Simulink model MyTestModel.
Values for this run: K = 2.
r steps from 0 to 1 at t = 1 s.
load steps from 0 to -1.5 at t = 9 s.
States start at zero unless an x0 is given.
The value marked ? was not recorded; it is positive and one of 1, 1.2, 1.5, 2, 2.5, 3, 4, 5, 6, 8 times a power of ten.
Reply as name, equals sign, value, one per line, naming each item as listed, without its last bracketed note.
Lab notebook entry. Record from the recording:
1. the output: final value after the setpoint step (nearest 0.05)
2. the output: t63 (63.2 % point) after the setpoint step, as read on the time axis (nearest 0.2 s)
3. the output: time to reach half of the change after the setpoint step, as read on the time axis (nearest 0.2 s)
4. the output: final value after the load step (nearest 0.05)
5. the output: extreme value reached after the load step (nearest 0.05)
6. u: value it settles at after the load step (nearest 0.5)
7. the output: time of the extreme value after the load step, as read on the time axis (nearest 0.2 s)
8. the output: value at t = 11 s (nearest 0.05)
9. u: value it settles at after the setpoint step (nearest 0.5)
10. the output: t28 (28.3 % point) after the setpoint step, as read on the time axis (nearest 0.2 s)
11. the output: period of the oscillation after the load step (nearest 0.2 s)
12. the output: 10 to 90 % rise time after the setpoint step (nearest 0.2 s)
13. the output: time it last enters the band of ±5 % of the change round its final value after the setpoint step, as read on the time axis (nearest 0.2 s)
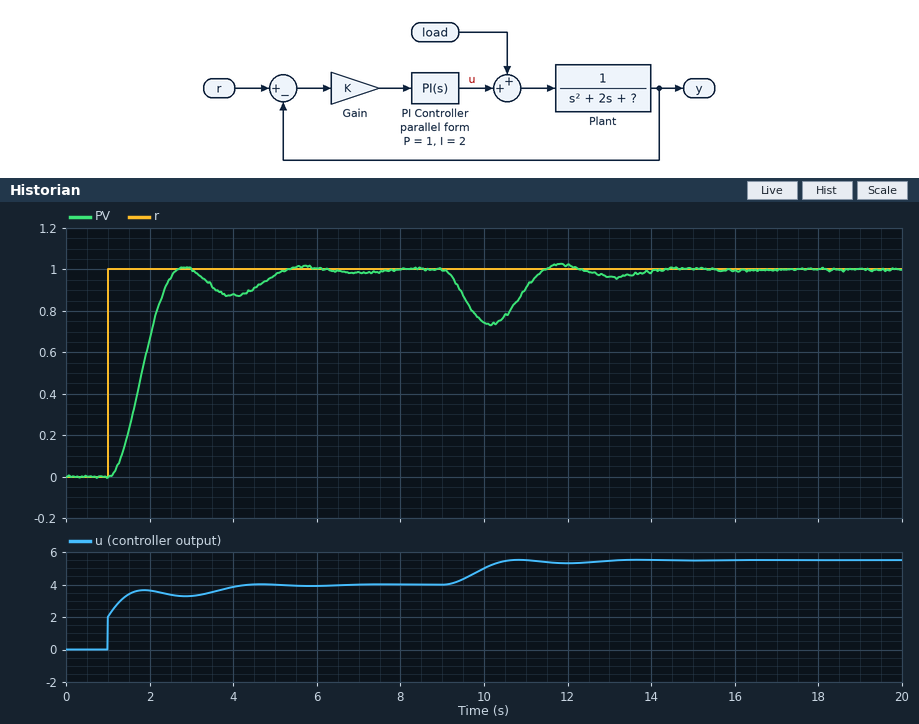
the output: final value after the setpoint step = 1.00
the output: t63 (63.2 % point) after the setpoint step, as read on the time axis = 2.0 s
the output: time to reach half of the change after the setpoint step, as read on the time axis = 1.8 s
the output: final value after the load step = 1.00
the output: extreme value reached after the load step = 0.75
u: value it settles at after the load step = 5.5
the output: time of the extreme value after the load step, as read on the time axis = 10.2 s
the output: value at t = 11 s = 0.90
u: value it settles at after the setpoint step = 4.0
the output: t28 (28.3 % point) after the setpoint step, as read on the time axis = 1.6 s
the output: period of the oscillation after the load step = 3.0 s
the output: 10 to 90 % rise time after the setpoint step = 1.0 s
the output: time it last enters the band of ±5 % of the change round its final value after the setpoint step, as read on the time axis = 4.8 s
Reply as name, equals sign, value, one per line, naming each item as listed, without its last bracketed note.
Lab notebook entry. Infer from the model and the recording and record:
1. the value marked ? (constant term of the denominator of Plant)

the value marked ? = 4
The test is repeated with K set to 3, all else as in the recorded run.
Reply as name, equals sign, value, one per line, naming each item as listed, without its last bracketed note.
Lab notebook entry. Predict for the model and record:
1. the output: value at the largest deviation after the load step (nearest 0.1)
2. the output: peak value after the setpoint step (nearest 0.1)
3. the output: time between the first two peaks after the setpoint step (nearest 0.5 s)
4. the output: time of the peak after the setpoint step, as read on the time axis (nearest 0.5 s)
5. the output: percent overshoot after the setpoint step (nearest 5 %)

the output: value at the largest deviation after the load step = 0.8
the output: peak value after the setpoint step = 1.2
the output: time between the first two peaks after the setpoint step = 2.5 s
the output: time of the peak after the setpoint step, as read on the time axis = 2.5 s
the output: percent overshoot after the setpoint step = 15 %
